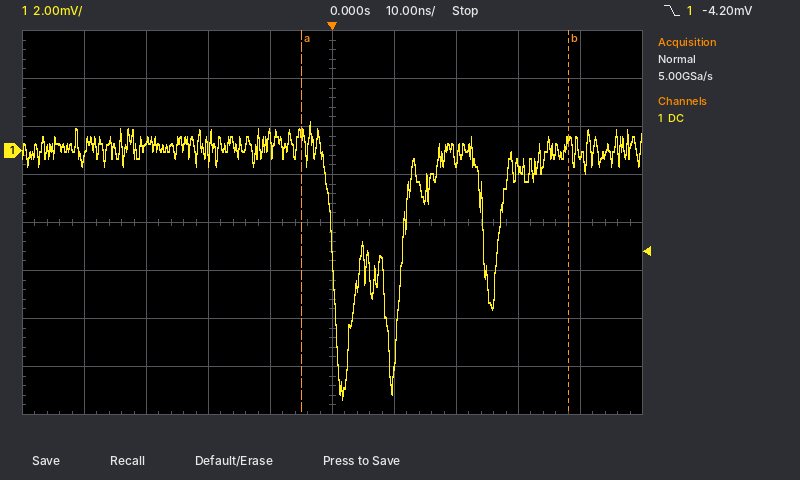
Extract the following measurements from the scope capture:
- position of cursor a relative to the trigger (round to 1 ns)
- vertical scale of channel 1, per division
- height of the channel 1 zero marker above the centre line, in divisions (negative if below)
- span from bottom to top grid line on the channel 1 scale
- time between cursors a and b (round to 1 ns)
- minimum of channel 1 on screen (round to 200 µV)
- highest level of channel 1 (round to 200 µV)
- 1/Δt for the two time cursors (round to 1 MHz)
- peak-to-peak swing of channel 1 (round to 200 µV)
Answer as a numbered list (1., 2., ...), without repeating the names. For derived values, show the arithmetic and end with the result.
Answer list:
1. -5 ns
2. 2 mV
3. +1.5 div
4. 16 mV
5. 43 ns
6. -10.4 mV
7. 1.2 mV
8. 1 / 43 ns ≈ 23 MHz
9. 1.2 mV − (-10.4 mV) = 11.6 mV
